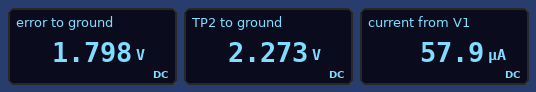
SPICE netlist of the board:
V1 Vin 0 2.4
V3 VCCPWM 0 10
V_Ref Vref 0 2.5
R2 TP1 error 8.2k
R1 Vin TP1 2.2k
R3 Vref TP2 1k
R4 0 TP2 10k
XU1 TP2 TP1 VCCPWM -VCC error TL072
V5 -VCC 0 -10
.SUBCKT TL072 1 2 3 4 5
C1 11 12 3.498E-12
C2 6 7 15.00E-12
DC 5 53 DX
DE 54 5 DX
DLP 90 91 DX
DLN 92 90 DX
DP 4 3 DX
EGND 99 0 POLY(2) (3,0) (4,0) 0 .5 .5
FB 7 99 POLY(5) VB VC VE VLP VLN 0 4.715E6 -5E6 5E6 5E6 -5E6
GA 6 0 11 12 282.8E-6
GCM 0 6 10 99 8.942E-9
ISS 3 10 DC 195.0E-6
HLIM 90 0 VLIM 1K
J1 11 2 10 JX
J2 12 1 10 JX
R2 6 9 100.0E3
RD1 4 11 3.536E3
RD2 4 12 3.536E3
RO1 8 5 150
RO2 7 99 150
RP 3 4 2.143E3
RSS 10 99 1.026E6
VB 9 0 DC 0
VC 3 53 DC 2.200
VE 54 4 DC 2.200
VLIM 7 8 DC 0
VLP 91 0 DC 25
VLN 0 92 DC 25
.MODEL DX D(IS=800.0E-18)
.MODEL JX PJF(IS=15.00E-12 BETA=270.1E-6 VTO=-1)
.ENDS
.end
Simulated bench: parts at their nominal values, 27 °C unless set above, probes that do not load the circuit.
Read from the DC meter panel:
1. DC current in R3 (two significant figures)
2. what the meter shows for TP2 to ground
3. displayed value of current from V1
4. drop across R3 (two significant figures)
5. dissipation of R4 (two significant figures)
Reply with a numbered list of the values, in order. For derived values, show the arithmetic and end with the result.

1. (2.5 V - 2.273 V) / 1 kΩ = 230 µA
2. 2.273 V
3. 57.9 µA
4. 2.5 V - 2.273 V = 230 mV
5. (2.273 V)^2 / 10 kΩ = 520 µW
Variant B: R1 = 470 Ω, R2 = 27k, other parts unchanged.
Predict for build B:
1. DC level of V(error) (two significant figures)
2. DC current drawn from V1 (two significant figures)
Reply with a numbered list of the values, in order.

1. -5.0 V
2. 270 µA
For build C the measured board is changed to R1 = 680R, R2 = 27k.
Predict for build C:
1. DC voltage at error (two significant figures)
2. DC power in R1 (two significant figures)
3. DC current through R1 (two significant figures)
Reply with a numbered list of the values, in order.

1. -2.8 V
2. 24 µW
3. 190 µA
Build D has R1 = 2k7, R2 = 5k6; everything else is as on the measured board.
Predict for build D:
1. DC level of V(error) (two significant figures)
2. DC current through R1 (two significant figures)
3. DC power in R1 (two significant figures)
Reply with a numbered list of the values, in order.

1. 2.0 V
2. 47 µA
3. 6.0 µW
